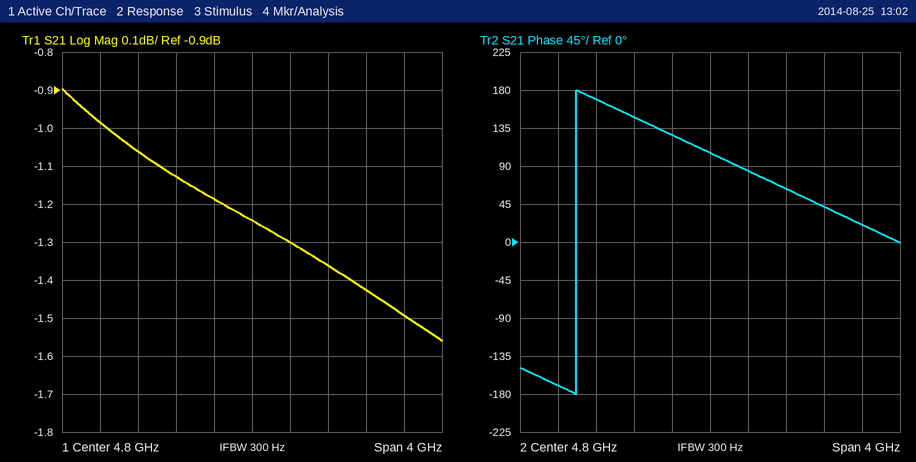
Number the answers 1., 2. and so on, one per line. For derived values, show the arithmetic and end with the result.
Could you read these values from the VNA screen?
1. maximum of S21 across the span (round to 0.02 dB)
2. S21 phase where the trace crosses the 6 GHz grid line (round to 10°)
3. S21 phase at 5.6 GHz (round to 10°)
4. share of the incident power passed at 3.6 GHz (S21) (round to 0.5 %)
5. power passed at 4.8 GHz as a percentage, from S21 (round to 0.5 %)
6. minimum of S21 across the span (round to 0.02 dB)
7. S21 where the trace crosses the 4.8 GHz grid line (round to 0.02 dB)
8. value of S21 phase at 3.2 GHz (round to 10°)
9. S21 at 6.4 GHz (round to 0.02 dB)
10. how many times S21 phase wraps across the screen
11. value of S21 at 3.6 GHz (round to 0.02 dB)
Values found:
1. -0.90 dB
2. 40°
3. 60°
4. 10^(-1.06/10) ≈ 78.3 %, so 78.5 % to the nearest 0.5 %
5. 10^(-1.24/10) ≈ 75.2 %, so 75.0 % to the nearest 0.5 %
6. -1.56 dB
7. -1.24 dB
8. -170°
9. -1.50 dB
10. 1
11. -1.06 dB
